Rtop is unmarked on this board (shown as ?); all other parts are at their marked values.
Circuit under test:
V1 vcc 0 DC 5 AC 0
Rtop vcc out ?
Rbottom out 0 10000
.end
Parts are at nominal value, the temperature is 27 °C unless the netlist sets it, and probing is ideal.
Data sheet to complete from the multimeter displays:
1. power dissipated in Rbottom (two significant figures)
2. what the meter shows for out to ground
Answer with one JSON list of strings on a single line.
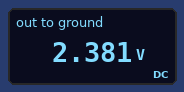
["570 µW", "2.381 V"]
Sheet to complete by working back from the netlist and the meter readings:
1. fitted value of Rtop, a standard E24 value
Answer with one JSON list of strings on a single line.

["11 kΩ"]
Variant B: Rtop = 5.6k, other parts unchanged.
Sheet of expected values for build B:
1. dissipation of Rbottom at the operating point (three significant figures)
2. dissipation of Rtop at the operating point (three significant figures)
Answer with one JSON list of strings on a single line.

["1.03 mW", "575 µW"]
